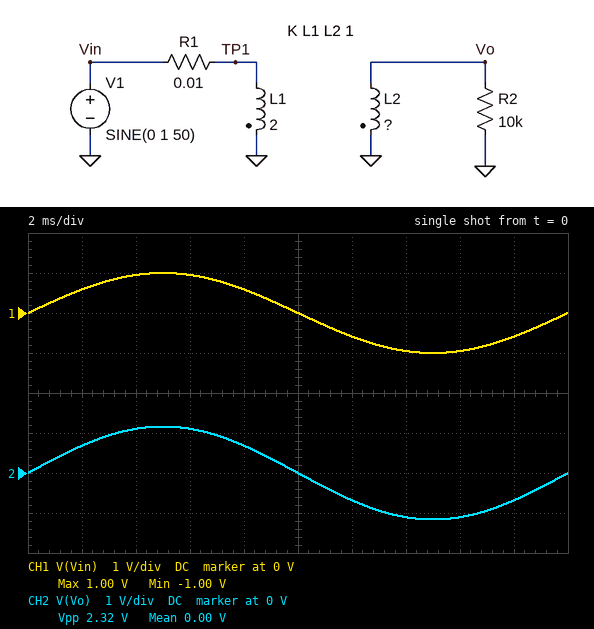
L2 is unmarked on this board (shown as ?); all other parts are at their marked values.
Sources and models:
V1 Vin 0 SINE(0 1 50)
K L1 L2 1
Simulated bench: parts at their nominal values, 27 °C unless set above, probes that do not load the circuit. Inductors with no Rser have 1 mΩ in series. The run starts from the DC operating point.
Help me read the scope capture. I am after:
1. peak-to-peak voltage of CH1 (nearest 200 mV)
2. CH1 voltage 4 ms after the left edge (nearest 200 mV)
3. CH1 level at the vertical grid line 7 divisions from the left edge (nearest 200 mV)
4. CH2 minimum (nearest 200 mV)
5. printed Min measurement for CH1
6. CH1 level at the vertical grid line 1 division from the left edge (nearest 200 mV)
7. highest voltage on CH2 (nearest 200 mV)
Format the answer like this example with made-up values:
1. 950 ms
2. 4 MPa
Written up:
1. 2.0 V
2. 1.0 V
3. -1.0 V
4. -1.2 V
5. -1.00 V
6. 600 mV
7. 1.2 V
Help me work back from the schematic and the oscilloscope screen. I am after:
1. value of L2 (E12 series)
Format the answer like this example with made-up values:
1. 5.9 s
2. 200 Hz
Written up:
1. 2.7 H
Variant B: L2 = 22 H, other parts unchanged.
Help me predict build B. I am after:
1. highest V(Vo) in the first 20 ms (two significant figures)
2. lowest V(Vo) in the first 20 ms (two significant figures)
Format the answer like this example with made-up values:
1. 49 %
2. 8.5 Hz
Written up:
1. 3.3 V
2. -3.3 V
